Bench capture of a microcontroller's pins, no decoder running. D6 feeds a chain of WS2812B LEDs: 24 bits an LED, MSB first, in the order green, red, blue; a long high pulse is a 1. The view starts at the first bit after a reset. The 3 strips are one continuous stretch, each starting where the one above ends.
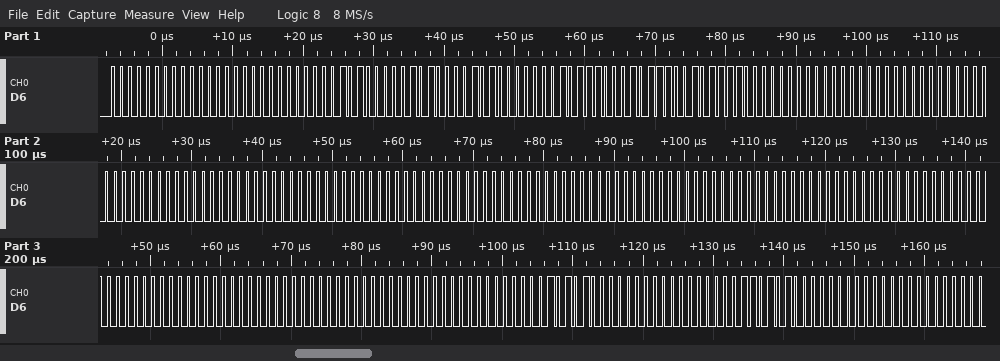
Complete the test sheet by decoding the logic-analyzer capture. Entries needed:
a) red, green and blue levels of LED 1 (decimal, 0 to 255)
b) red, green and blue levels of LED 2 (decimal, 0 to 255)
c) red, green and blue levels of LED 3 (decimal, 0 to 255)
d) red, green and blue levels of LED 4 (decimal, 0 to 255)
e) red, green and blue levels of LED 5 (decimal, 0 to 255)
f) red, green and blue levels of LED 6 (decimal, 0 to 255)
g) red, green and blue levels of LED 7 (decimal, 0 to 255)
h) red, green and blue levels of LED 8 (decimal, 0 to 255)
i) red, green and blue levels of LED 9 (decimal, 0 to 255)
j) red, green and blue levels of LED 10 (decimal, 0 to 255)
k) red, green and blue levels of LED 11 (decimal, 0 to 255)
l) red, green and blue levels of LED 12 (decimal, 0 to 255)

0, 0, 0
40, 40, 80
23, 23, 47
0, 0, 0
0, 0, 0
0, 0, 0
0, 0, 0
0, 0, 0
0, 0, 0
0, 0, 0
21, 0, 0
106, 0, 0
